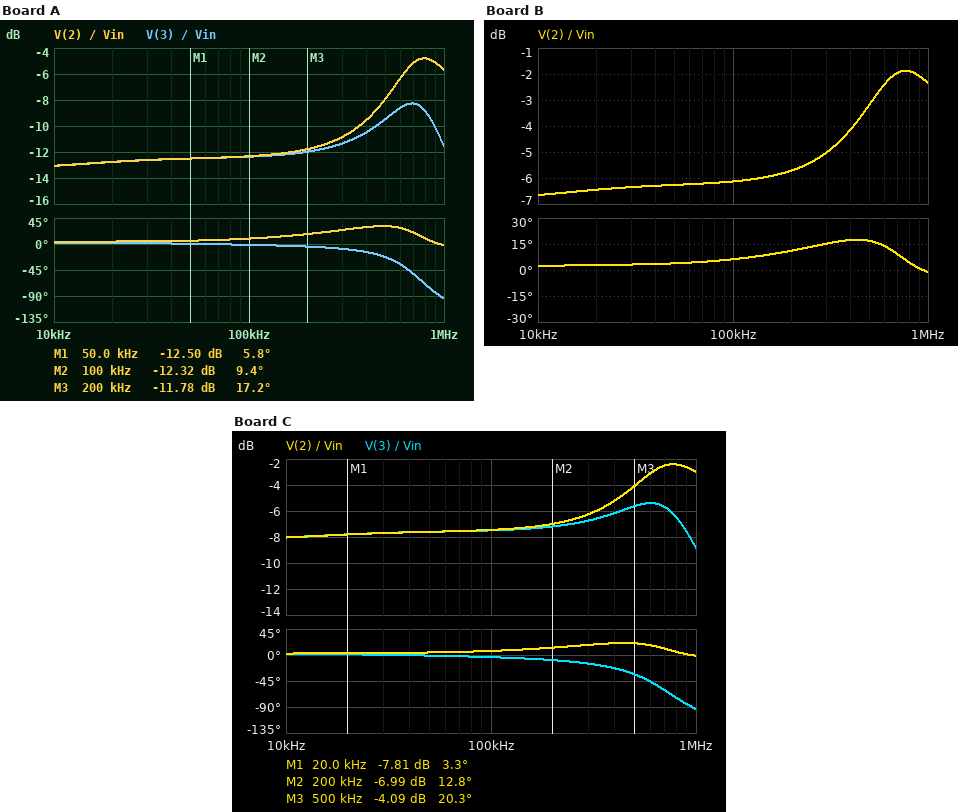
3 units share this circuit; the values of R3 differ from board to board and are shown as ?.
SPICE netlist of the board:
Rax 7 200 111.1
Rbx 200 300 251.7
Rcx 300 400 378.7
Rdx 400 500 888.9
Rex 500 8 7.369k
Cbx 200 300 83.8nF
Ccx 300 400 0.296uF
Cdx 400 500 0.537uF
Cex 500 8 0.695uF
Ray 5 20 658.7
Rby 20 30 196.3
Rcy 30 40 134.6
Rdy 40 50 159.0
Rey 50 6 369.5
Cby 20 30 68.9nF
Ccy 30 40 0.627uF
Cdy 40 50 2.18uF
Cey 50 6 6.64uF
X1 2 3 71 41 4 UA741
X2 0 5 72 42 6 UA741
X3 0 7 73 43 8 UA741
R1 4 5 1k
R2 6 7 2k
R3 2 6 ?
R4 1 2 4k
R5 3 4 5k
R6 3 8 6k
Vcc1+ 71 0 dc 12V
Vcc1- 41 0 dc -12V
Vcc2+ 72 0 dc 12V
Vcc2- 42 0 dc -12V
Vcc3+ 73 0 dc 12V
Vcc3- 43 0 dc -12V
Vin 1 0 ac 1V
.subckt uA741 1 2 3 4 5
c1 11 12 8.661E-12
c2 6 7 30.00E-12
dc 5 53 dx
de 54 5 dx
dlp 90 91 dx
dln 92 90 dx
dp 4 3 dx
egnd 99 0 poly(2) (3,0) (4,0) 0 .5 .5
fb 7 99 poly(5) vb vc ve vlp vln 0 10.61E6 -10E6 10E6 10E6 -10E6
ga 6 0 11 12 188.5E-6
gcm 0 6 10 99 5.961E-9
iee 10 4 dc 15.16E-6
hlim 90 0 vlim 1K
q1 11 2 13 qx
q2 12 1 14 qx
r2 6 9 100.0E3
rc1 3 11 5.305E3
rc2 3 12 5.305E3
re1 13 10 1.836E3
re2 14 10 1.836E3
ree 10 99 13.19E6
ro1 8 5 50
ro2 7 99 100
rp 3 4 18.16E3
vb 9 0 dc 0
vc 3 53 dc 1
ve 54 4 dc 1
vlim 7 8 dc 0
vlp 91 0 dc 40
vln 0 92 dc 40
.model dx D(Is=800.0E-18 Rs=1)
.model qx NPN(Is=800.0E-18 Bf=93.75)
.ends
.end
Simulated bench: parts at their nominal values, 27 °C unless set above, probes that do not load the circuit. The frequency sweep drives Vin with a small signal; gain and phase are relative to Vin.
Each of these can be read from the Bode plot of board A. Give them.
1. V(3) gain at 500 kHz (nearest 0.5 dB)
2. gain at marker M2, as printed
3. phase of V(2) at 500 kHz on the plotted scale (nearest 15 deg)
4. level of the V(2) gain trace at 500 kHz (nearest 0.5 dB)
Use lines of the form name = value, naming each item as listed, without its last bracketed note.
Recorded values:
V(3) gain at 500 kHz = -9.5 dB
gain at marker M2, as printed = -12.32 dB
phase of V(2) at 500 kHz on the plotted scale = 30 deg
level of the V(2) gain trace at 500 kHz = -8.0 dB
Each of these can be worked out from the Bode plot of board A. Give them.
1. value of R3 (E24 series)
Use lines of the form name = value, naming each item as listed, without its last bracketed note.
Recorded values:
value of R3 = 2.7 kΩ
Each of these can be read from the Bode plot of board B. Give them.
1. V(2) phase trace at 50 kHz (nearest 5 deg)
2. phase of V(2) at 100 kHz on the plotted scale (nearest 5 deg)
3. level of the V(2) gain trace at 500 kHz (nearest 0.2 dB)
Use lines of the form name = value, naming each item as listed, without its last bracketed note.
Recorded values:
V(2) phase trace at 50 kHz = 5 deg
phase of V(2) at 100 kHz on the plotted scale = 5 deg
level of the V(2) gain trace at 500 kHz = -3.2 dB
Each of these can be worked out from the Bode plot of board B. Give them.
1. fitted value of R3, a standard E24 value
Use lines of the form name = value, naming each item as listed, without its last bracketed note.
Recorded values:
fitted value of R3, a standard E24 value = 8.2 kΩ
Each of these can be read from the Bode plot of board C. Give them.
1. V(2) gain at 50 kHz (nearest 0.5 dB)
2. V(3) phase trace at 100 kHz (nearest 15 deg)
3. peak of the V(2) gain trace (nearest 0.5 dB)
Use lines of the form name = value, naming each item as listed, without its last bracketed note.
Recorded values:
V(2) gain at 50 kHz = -7.5 dB
V(3) phase trace at 100 kHz = 0 deg
peak of the V(2) gain trace = -2.5 dB
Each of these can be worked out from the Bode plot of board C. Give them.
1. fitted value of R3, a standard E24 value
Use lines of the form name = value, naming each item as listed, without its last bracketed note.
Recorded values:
fitted value of R3, a standard E24 value = 6.2 kΩ
